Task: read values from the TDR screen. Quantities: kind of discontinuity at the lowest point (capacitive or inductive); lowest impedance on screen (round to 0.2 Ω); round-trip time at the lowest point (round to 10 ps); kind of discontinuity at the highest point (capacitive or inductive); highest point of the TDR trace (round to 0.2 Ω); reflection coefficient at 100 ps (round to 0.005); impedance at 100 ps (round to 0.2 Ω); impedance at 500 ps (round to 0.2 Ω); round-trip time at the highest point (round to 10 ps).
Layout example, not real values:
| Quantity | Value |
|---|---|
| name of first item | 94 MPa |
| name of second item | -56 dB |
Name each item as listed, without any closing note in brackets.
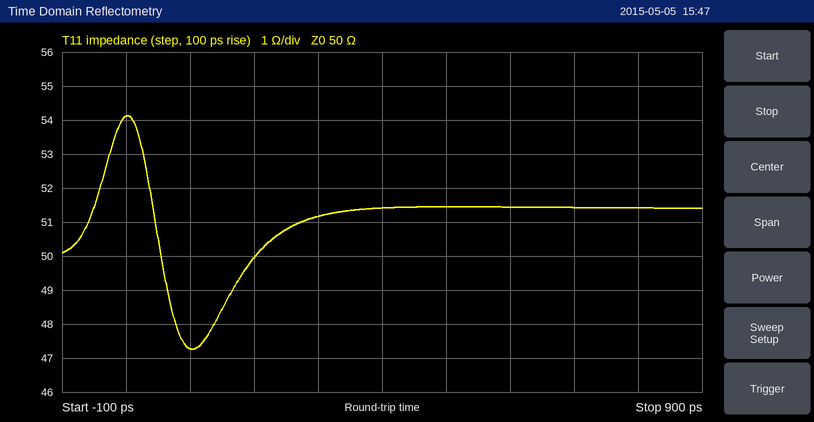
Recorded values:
| Quantity | Value |
|---|---|
| kind of discontinuity at the lowest point | capacitive |
| lowest impedance on screen | 47.2 Ω |
| round-trip time at the lowest point | 100 ps |
| kind of discontinuity at the highest point | inductive |
| highest point of the TDR trace | 54.2 Ω |
| reflection coefficient at 100 ps | -0.030 |
| impedance at 100 ps | 47.2 Ω |
| impedance at 500 ps | 51.4 Ω |
| round-trip time at the highest point | 0 ps |
